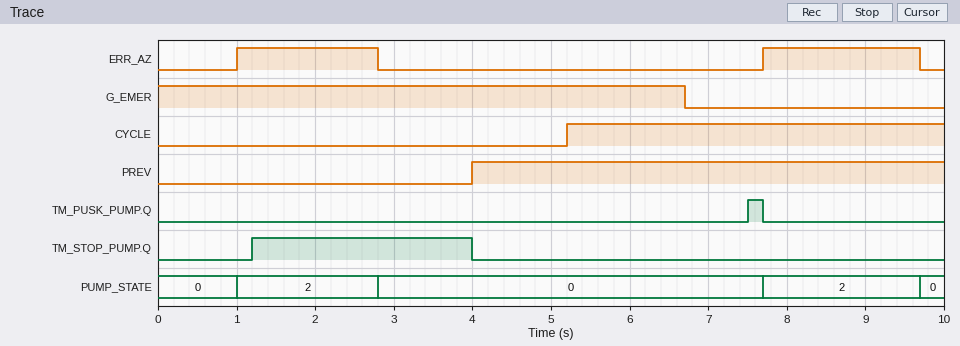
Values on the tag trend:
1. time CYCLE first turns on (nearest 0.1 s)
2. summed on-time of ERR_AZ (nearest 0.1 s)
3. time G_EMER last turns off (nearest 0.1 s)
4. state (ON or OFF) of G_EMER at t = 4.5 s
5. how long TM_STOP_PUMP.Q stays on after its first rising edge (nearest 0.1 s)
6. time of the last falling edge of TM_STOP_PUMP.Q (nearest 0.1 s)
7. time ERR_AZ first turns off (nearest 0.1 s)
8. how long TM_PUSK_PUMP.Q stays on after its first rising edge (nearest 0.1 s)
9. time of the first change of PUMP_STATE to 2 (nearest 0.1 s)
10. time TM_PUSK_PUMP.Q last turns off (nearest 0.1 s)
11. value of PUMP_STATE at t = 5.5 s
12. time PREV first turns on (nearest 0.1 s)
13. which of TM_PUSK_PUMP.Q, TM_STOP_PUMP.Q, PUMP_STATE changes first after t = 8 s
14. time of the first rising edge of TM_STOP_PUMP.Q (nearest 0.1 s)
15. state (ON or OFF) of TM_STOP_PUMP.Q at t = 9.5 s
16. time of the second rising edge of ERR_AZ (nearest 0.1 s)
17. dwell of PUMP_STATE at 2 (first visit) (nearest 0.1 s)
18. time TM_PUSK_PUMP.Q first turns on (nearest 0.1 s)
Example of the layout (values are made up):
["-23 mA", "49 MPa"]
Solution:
["5.2 s", "3.8 s", "6.7 s", "ON", "2.8 s", "4.0 s", "2.8 s", "0.2 s", "1.0 s", "7.7 s", "0", "4.0 s", "PUMP_STATE", "1.2 s", "OFF", "7.7 s", "1.8 s", "7.5 s"]
